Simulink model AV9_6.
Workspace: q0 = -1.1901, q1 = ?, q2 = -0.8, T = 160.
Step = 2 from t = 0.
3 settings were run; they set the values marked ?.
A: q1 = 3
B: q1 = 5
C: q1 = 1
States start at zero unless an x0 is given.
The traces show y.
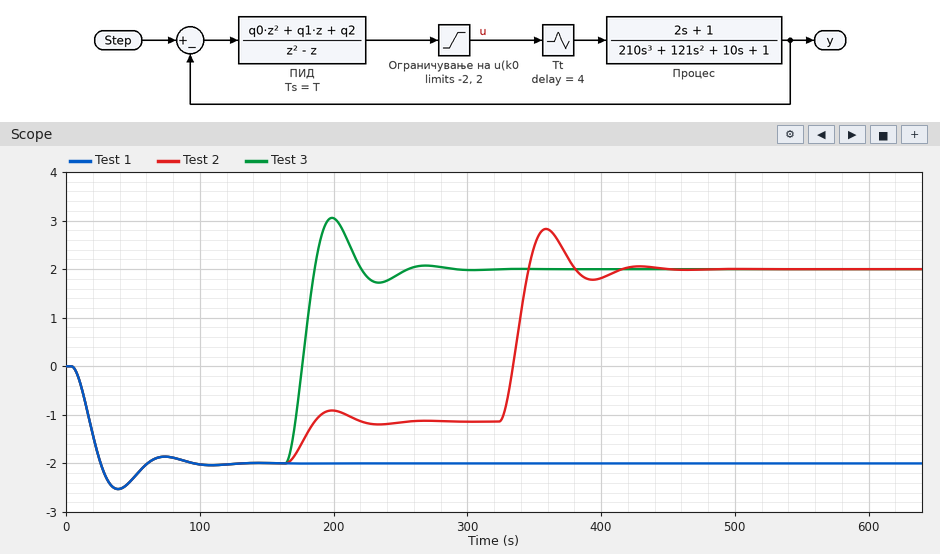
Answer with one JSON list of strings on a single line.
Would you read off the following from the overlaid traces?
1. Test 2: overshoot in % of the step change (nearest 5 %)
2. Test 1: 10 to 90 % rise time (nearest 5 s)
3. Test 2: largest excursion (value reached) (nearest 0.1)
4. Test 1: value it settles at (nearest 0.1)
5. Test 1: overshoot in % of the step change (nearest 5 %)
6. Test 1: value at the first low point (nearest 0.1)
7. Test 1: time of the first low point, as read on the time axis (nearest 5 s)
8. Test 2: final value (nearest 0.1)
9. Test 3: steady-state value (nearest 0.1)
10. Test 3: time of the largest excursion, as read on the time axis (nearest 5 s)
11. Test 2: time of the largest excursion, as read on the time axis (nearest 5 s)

["40 %", "15 s", "2.8", "-2.0", "25 %", "-2.5", "40 s", "2.0", "2.0", "200 s", "360 s"]
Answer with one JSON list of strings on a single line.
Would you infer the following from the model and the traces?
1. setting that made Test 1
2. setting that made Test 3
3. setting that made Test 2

["C", "B", "A"]
